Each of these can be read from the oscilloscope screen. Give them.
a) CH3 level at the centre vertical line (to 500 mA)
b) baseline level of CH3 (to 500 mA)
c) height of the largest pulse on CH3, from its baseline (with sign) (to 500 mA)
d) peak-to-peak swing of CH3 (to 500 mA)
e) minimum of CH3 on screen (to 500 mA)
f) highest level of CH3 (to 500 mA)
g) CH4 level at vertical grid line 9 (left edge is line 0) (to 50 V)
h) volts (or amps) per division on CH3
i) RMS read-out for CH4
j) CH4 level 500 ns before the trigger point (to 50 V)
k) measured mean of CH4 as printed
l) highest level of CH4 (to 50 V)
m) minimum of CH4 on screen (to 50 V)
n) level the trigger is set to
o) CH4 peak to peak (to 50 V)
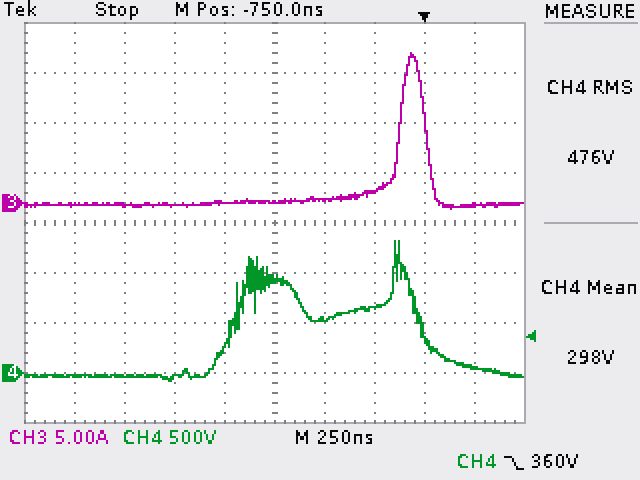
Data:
0.0 A
0.0 A
+15.0 A
15.5 A
-500 mA
15.0 A
50 V
5 A
476 V
550 V
298 V
1.30 kV
-100 V
360 V
1.40 kV
